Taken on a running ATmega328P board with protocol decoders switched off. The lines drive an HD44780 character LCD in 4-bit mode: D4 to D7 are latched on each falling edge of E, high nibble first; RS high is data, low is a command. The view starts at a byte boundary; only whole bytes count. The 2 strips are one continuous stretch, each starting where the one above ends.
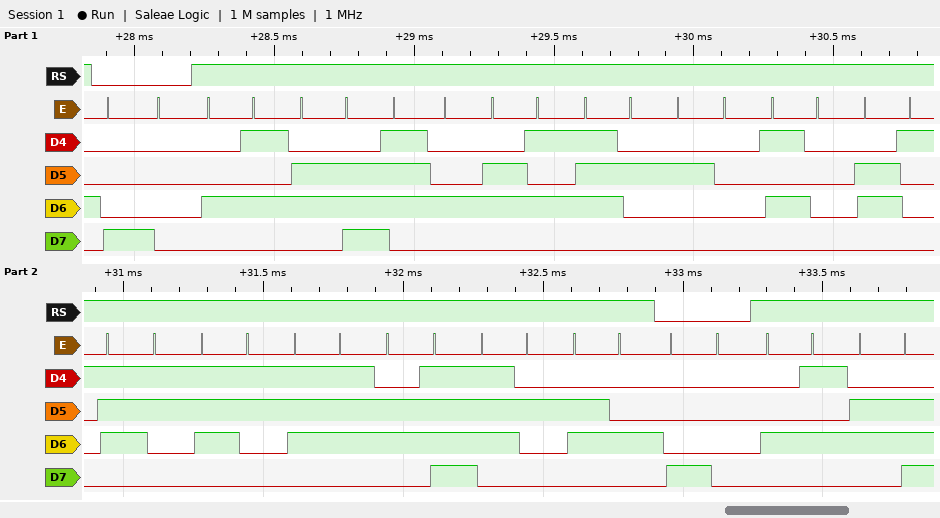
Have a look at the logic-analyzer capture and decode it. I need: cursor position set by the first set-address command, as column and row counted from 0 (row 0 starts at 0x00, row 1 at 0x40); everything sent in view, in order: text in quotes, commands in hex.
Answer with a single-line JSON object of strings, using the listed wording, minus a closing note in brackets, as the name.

{"cursor position set by the first set-address command, as column and row counted from 0": "column 0, row 0", "everything sent in view, in order: text in quotes, commands in hex": "0x80 \"Enter Password\" 0x80 \"En\""}
